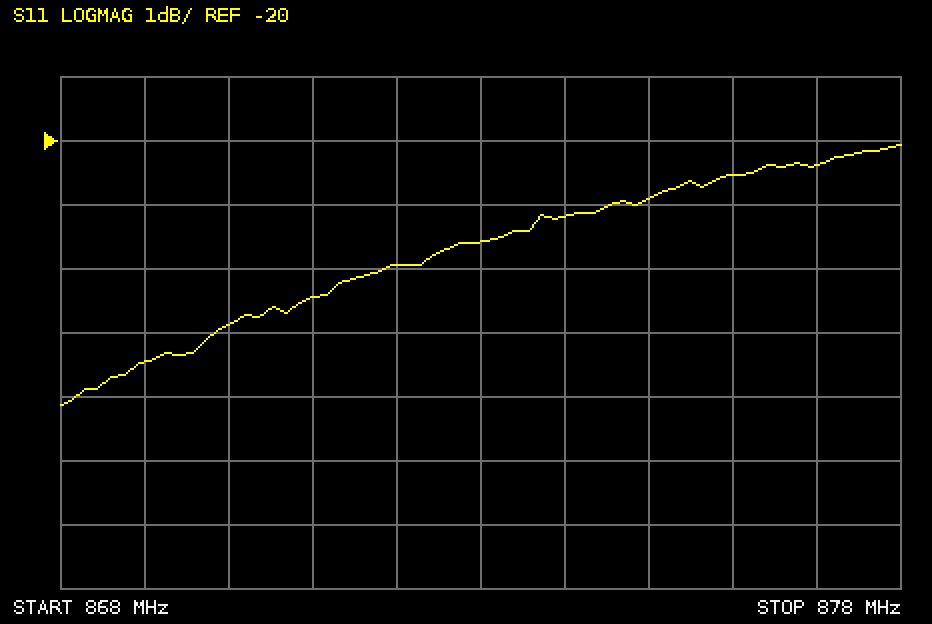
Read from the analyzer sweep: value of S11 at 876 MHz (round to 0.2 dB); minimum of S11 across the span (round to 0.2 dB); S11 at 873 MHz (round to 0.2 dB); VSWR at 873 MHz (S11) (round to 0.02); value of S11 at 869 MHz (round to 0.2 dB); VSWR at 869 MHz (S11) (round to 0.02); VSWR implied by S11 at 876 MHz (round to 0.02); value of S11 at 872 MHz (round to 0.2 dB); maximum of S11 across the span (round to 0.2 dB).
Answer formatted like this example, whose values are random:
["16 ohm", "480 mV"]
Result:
["-20.6 dB", "-24.2 dB", "-21.6 dB", "1.18", "-23.4 dB", "1.14", "1.20", "-22.0 dB", "-20.0 dB"]
